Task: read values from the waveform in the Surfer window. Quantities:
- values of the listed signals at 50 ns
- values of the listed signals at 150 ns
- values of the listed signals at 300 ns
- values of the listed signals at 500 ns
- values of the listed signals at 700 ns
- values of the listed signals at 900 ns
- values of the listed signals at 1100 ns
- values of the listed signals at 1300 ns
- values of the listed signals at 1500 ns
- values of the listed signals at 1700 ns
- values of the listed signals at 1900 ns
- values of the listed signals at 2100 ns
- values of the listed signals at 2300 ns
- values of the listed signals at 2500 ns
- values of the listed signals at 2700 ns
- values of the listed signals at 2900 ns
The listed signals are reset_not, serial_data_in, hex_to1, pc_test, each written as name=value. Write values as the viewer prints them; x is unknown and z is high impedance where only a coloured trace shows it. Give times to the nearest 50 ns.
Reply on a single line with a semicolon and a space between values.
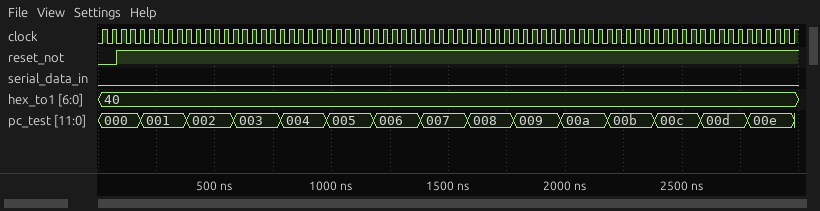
reset_not=0, serial_data_in=0, hex_to1=40, pc_test=000; reset_not=1, serial_data_in=0, hex_to1=40, pc_test=000; reset_not=1, serial_data_in=0, hex_to1=40, pc_test=001; reset_not=1, serial_data_in=0, hex_to1=40, pc_test=002; reset_not=1, serial_data_in=0, hex_to1=40, pc_test=003; reset_not=1, serial_data_in=0, hex_to1=40, pc_test=004; reset_not=1, serial_data_in=0, hex_to1=40, pc_test=005; reset_not=1, serial_data_in=0, hex_to1=40, pc_test=006; reset_not=1, serial_data_in=0, hex_to1=40, pc_test=007; reset_not=1, serial_data_in=0, hex_to1=40, pc_test=008; reset_not=1, serial_data_in=0, hex_to1=40, pc_test=009; reset_not=1, serial_data_in=0, hex_to1=40, pc_test=00a; reset_not=1, serial_data_in=0, hex_to1=40, pc_test=00b; reset_not=1, serial_data_in=0, hex_to1=40, pc_test=00c; reset_not=1, serial_data_in=0, hex_to1=40, pc_test=00d; reset_not=1, serial_data_in=0, hex_to1=40, pc_test=00e
